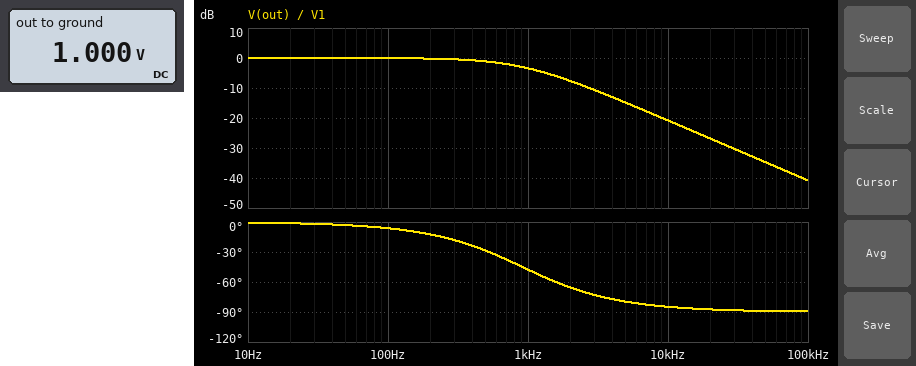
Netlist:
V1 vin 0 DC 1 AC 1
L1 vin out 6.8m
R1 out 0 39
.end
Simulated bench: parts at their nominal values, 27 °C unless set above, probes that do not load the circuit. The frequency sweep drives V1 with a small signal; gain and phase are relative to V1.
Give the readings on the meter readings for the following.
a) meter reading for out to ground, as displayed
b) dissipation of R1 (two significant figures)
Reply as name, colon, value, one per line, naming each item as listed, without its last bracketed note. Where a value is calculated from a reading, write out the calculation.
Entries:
meter reading for out to ground, as displayed: 1.000 V
dissipation of R1: (1 V)^2 / 39 Ω = 26 mW
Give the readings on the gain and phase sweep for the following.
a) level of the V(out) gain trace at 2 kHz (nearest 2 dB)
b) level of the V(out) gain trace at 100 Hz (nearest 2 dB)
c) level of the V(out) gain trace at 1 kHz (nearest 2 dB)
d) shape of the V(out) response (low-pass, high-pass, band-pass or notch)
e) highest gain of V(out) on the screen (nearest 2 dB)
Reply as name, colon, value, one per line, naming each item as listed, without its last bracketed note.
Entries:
level of the V(out) gain trace at 2 kHz: -8 dB
level of the V(out) gain trace at 100 Hz: 0 dB
level of the V(out) gain trace at 1 kHz: -4 dB
shape of the V(out) response: low-pass
highest gain of V(out) on the screen: 0 dB
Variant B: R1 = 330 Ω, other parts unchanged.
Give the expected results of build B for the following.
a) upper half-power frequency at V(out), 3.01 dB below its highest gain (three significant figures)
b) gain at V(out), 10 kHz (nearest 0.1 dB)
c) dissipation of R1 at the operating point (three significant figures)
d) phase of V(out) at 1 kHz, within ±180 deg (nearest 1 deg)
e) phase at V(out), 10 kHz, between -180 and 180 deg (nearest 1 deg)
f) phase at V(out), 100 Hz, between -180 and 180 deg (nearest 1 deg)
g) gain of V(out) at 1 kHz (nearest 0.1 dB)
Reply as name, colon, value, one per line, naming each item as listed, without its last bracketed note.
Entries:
upper half-power frequency at V(out), 3.01 dB below its highest gain: 7.72 kHz
gain at V(out), 10 kHz: -4.3 dB
dissipation of R1 at the operating point: 3.03 mW
phase of V(out) at 1 kHz, within ±180 deg: -7 deg
phase at V(out), 10 kHz, between -180 and 180 deg: -52 deg
phase at V(out), 100 Hz, between -180 and 180 deg: -1 deg
gain of V(out) at 1 kHz: -0.1 dB
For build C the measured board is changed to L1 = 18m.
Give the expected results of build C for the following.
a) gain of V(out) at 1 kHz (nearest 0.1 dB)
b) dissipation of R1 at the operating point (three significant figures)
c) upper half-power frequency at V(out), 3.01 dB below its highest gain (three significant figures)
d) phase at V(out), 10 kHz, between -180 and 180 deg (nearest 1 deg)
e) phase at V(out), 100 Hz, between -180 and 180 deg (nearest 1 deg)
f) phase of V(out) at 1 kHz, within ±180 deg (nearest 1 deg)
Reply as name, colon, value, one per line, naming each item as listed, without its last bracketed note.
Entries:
gain of V(out) at 1 kHz: -9.7 dB
dissipation of R1 at the operating point: 25.6 mW
upper half-power frequency at V(out), 3.01 dB below its highest gain: 345 Hz
phase at V(out), 10 kHz, between -180 and 180 deg: -88 deg
phase at V(out), 100 Hz, between -180 and 180 deg: -16 deg
phase of V(out) at 1 kHz, within ±180 deg: -71 deg
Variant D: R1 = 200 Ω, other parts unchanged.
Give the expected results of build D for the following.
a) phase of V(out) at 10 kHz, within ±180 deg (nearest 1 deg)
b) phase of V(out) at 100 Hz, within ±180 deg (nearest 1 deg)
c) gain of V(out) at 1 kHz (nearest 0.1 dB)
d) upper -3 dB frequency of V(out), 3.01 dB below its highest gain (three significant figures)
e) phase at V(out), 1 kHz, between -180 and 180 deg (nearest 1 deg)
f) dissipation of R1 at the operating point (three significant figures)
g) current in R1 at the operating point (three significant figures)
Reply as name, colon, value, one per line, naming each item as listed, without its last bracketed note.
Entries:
phase of V(out) at 10 kHz, within ±180 deg: -65 deg
phase of V(out) at 100 Hz, within ±180 deg: -1 deg
gain of V(out) at 1 kHz: -0.2 dB
upper -3 dB frequency of V(out), 3.01 dB below its highest gain: 4.68 kHz
phase at V(out), 1 kHz, between -180 and 180 deg: -12 deg
dissipation of R1 at the operating point: 5.00 mW
current in R1 at the operating point: 5.00 mA
